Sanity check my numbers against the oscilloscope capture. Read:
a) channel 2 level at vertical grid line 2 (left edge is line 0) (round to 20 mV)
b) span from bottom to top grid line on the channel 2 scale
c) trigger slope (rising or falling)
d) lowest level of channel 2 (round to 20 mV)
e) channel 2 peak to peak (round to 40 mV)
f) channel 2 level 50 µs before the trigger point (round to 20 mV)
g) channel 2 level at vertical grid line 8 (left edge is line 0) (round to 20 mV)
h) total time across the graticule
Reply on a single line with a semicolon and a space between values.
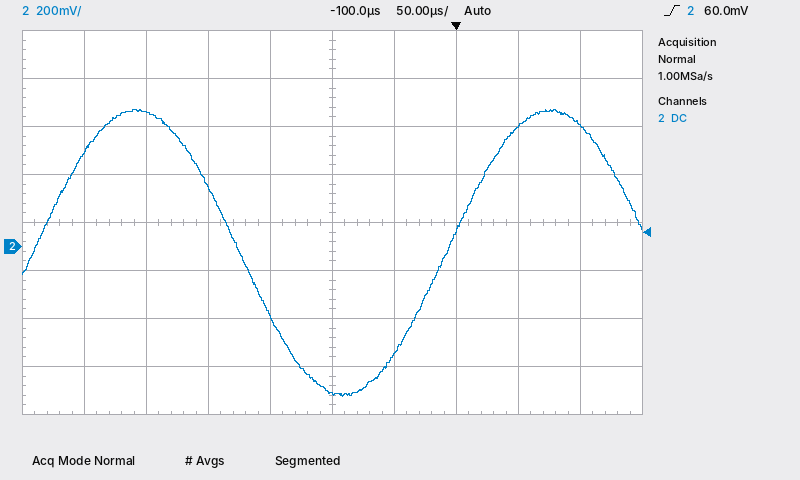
560 mV; 1.6 V; rising; -620 mV; 1.20 V; -440 mV; 500 mV; 500 µs
